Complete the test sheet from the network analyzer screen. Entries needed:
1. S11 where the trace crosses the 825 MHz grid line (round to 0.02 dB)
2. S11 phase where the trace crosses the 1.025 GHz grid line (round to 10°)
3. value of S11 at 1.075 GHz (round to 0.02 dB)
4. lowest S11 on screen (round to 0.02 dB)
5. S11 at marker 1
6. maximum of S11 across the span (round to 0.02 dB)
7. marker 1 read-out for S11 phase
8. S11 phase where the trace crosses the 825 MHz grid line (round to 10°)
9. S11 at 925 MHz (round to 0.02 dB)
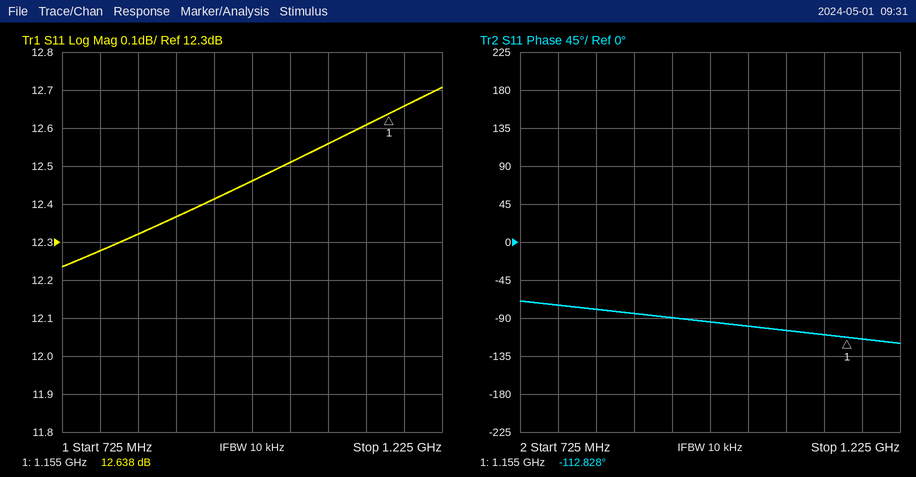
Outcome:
12.32 dB
-100°
12.56 dB
12.24 dB
12.638 dB
12.70 dB
-112.828°
-80°
12.42 dB
